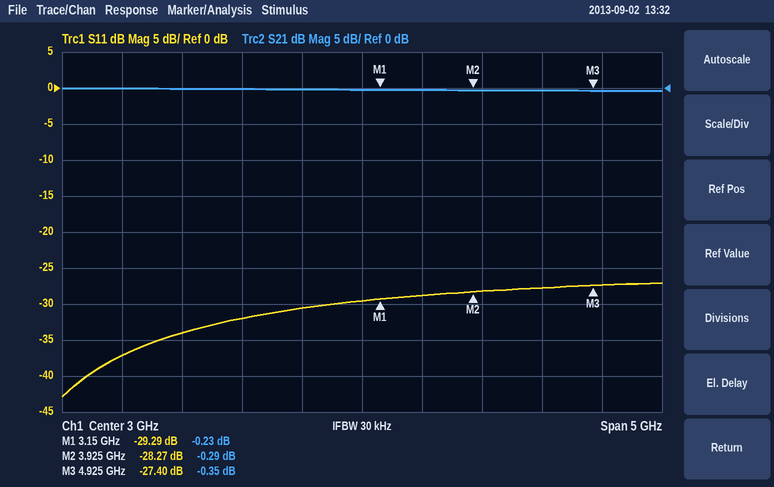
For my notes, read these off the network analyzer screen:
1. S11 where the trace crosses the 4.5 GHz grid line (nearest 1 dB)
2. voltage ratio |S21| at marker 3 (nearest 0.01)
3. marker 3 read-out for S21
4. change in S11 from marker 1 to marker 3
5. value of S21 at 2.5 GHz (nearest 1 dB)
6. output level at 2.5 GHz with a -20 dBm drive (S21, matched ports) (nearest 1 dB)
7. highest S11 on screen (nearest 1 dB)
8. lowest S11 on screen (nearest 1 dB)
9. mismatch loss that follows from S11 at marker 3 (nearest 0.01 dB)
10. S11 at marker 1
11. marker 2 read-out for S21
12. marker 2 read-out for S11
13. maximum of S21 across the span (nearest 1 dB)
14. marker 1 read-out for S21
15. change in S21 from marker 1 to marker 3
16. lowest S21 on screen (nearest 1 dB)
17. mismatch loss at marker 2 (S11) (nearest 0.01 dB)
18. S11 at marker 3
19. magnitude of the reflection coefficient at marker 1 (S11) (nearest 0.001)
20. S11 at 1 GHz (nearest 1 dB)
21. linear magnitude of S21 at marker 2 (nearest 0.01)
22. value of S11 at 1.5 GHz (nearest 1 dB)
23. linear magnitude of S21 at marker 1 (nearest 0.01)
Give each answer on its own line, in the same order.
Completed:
-28 dB
0.96
-0.35 dB
1.89 dB
0 dB
-20 dBm
-27 dB
-43 dB
0.01 dB
-29.29 dB
-0.29 dB
-28.27 dB
0 dB
-0.23 dB
-0.12 dB
0 dB
0.01 dB
-27.40 dB
0.034
-37 dB
0.97
-34 dB
0.97
